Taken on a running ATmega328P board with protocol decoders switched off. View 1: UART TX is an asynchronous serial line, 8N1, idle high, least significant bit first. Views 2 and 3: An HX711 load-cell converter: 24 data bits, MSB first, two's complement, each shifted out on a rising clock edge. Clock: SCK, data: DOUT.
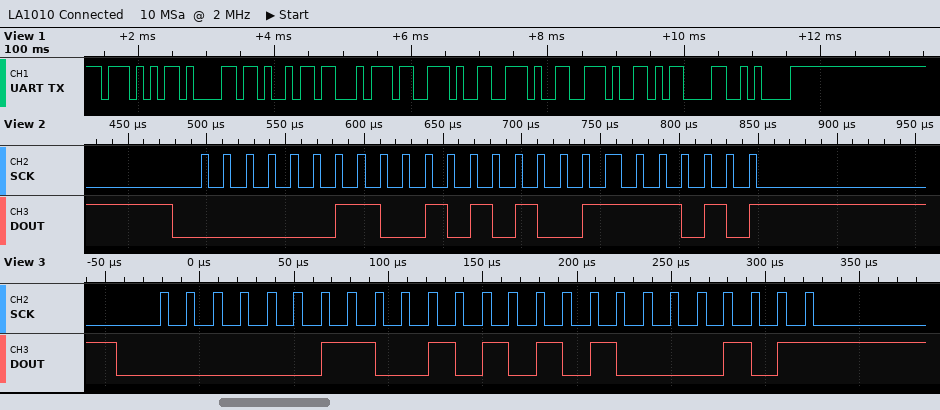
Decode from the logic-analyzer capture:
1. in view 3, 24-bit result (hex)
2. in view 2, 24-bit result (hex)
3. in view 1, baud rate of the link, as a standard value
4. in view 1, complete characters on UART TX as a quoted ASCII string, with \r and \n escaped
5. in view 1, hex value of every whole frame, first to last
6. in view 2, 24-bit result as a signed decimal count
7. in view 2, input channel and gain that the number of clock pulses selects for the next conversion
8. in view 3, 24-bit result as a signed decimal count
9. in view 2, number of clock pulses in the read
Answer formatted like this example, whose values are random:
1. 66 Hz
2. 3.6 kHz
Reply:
1. 0x032A85
2. 0x032A7A
3. 9600 baud
4. "Wait...\r\n"
5. 57 61 69 74 2E 2E 2E 0D 0A
6. 207482
7. channel A, gain 128
8. 207493
9. 25
